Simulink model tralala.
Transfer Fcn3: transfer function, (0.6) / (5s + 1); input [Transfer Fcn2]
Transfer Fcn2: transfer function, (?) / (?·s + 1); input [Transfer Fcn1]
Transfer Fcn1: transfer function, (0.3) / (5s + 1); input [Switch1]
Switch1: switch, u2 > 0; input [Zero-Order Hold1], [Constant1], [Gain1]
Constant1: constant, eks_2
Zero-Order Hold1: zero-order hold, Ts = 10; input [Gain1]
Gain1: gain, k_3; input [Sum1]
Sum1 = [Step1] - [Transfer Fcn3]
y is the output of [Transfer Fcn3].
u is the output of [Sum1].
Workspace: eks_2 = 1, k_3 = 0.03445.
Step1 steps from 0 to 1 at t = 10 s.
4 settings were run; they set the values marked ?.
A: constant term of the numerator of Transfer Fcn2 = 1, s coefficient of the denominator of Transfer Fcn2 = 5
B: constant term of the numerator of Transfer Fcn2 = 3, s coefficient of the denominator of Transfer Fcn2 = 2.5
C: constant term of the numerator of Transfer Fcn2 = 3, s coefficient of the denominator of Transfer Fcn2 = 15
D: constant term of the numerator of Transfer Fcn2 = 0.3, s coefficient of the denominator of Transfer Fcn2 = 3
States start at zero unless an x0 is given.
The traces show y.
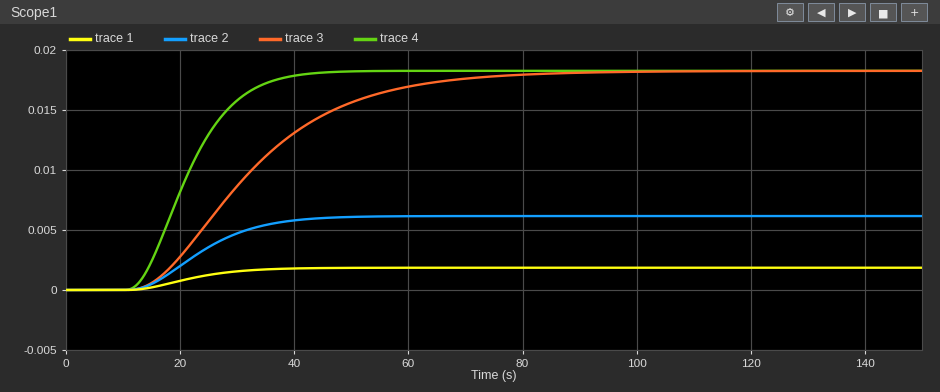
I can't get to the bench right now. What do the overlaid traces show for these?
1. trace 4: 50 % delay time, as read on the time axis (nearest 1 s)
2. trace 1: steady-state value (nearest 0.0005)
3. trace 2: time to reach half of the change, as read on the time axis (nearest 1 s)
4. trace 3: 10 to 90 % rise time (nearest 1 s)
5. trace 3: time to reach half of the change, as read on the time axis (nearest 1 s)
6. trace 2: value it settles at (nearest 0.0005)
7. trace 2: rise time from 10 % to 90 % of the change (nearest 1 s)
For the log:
21 s
0.0020
23 s
37 s
31 s
0.0060
21 s
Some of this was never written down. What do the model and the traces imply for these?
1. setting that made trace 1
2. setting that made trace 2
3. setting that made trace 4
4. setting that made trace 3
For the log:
D
A
B
C
